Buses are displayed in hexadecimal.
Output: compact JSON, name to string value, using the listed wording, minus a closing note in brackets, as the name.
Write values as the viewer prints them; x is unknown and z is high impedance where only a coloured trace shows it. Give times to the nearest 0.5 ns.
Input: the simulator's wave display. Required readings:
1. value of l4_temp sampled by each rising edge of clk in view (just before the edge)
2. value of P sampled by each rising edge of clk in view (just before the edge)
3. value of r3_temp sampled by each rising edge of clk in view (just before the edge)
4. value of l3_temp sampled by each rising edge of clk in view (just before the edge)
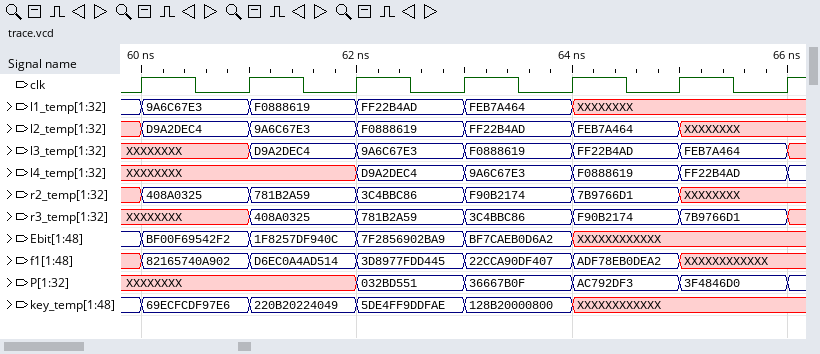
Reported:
{"value of l4_temp sampled by each rising edge of clk in view": "XXXXXXXX, XXXXXXXX, XXXXXXXX, D9A2DEC4, 9A6C67E3, F0888619, FF22B4AD", "value of P sampled by each rising edge of clk in view": "XXXXXXXX, XXXXXXXX, XXXXXXXX, 032BD551, 36667B0F, AC792DF3, 3F4846D0", "value of r3_temp sampled by each rising edge of clk in view": "XXXXXXXX, XXXXXXXX, 408A0325, 781B2A59, 3C4BBC86, F90B2174, 7B9766D1", "value of l3_temp sampled by each rising edge of clk in view": "XXXXXXXX, XXXXXXXX, D9A2DEC4, 9A6C67E3, F0888619, FF22B4AD, FEB7A464"}
